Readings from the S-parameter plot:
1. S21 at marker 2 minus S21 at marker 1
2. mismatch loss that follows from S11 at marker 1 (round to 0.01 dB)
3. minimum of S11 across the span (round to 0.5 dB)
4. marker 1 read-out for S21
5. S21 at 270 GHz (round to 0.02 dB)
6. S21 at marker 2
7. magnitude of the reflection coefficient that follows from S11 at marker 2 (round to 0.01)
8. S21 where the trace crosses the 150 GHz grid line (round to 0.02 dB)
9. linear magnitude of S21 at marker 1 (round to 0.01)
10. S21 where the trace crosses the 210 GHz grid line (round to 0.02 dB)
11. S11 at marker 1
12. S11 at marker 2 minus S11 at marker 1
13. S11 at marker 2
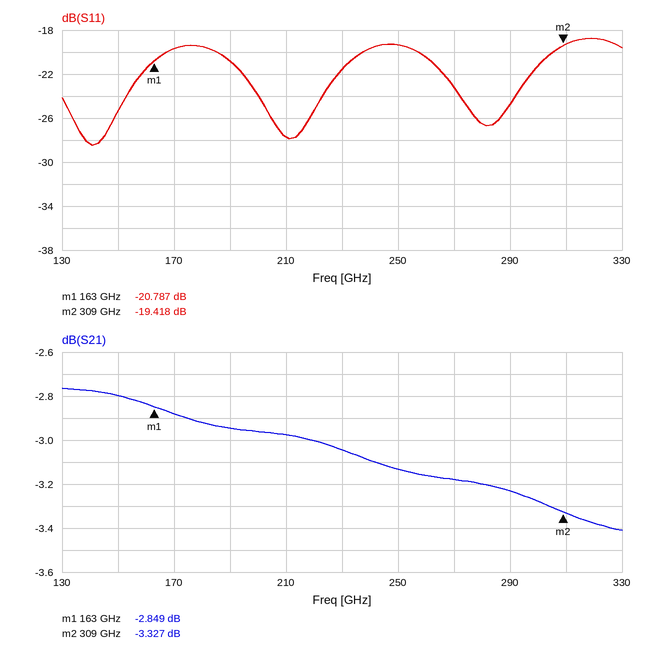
-0.478 dB
0.04 dB
-28.5 dB
-2.849 dB
-3.18 dB
-3.327 dB
0.11
-2.80 dB
0.72
-2.98 dB
-20.787 dB
1.369 dB
-19.418 dB
